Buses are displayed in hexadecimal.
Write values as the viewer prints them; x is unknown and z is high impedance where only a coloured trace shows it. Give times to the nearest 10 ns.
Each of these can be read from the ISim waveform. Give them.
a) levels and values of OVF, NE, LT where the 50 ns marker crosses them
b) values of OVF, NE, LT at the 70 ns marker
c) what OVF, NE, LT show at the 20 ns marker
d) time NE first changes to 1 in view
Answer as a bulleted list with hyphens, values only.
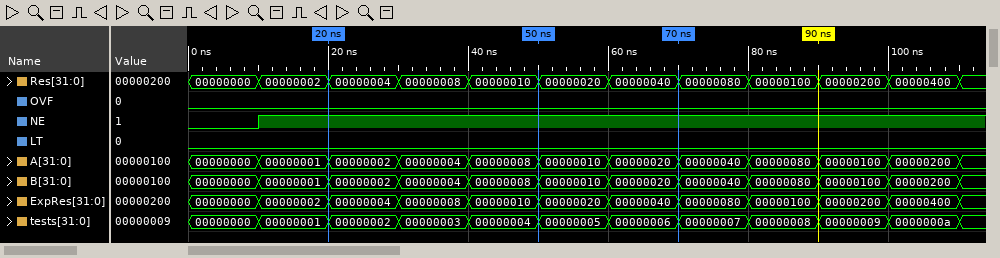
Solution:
- OVF=0, NE=1, LT=0
- OVF=0, NE=1, LT=0
- OVF=0, NE=1, LT=0
- 10 ns
